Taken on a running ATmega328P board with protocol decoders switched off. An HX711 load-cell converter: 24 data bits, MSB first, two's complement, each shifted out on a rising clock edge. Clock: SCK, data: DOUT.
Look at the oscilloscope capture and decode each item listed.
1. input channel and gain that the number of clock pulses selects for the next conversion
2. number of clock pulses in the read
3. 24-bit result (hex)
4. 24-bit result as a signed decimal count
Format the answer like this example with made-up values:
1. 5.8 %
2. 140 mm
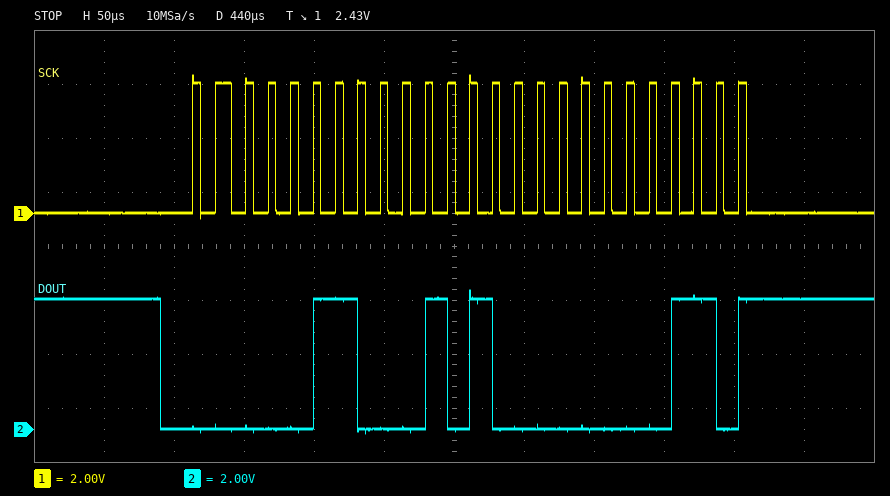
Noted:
1. channel A, gain 128
2. 25
3. 0x062806
4. 403462
